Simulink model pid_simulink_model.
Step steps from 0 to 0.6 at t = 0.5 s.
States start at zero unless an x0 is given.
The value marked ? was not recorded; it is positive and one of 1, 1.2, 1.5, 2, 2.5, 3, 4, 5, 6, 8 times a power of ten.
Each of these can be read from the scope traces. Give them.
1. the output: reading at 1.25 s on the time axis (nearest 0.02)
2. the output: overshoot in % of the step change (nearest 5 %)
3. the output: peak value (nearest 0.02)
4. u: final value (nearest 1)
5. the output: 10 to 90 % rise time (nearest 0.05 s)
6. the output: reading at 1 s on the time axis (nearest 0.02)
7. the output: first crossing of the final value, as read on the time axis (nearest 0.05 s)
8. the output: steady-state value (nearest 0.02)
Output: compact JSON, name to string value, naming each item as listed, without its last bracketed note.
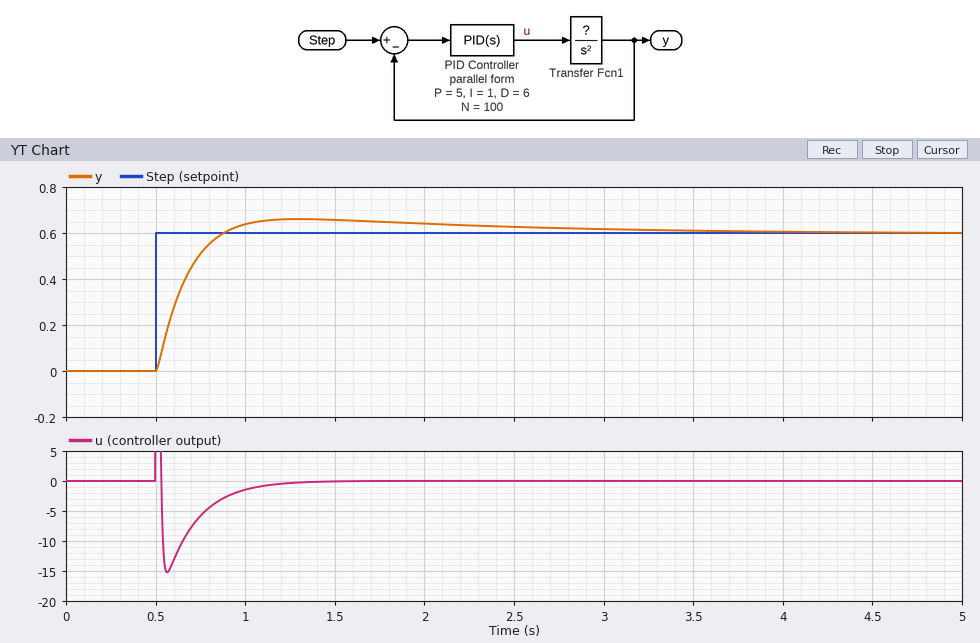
{"the output: reading at 1.25 s on the time axis": "0.66", "the output: overshoot in % of the step change": "10 %", "the output: peak value": "0.66", "u: final value": "0", "the output: 10 to 90 % rise time": "0.25 s", "the output: reading at 1 s on the time axis": "0.64", "the output: first crossing of the final value, as read on the time axis": "0.90 s", "the output: steady-state value": "0.60"}
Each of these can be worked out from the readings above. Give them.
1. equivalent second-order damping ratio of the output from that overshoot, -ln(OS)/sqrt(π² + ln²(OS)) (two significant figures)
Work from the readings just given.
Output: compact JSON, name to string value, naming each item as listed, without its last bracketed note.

{"equivalent second-order damping ratio of the output from that overshoot, -ln(OS)/sqrt(π² + ln²(OS))": "0.59"}
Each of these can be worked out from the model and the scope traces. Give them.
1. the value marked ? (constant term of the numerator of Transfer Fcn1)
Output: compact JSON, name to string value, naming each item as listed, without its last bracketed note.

{"the value marked ?": "1"}
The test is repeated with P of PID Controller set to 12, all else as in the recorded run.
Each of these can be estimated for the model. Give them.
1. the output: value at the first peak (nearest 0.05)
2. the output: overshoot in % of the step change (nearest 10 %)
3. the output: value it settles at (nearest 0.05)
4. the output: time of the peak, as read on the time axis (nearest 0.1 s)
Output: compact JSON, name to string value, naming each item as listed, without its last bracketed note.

{"the output: value at the first peak": "0.70", "the output: overshoot in % of the step change": "20 %", "the output: value it settles at": "0.60", "the output: time of the peak, as read on the time axis": "1.1 s"}
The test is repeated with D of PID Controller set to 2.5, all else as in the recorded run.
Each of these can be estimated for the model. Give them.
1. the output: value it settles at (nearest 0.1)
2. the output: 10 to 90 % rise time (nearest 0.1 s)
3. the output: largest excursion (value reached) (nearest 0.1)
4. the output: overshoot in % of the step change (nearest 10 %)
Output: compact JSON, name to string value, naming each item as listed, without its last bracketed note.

{"the output: value it settles at": "0.6", "the output: 10 to 90 % rise time": "0.4 s", "the output: largest excursion (value reached)": "0.8", "the output: overshoot in % of the step change": "30 %"}
